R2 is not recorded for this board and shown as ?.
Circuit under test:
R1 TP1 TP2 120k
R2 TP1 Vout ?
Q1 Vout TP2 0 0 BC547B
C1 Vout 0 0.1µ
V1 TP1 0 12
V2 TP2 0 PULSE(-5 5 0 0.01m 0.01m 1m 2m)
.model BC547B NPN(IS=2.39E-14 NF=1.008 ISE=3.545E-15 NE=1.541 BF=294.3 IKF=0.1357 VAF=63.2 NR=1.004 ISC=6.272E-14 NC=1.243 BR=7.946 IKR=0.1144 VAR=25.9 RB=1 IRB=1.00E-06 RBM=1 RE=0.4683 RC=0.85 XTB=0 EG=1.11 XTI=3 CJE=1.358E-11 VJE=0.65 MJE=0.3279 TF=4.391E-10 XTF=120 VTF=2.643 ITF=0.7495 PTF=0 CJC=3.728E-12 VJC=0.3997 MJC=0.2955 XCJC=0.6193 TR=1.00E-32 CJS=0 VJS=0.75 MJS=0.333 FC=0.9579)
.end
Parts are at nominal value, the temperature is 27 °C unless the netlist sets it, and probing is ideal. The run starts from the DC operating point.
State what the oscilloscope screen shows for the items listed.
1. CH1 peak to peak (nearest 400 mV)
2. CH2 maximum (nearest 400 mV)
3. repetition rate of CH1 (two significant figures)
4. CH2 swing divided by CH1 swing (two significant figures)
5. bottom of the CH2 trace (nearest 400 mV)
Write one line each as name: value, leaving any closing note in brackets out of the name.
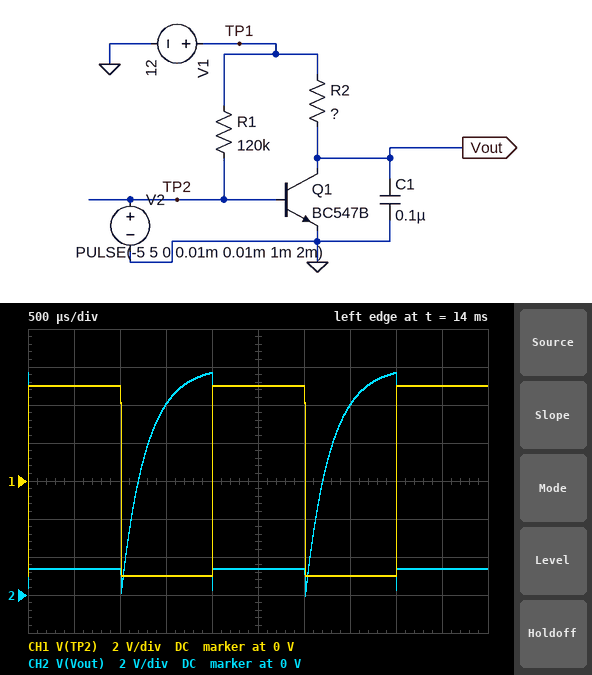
CH1 peak to peak: 10.0 V
CH2 maximum: 11.6 V
repetition rate of CH1: 500 Hz
CH2 swing divided by CH1 swing: 1.2
bottom of the CH2 trace: 0 V
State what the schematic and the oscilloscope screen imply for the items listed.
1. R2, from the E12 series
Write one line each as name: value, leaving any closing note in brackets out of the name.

R2, from the E12 series: 2.7 kΩ
